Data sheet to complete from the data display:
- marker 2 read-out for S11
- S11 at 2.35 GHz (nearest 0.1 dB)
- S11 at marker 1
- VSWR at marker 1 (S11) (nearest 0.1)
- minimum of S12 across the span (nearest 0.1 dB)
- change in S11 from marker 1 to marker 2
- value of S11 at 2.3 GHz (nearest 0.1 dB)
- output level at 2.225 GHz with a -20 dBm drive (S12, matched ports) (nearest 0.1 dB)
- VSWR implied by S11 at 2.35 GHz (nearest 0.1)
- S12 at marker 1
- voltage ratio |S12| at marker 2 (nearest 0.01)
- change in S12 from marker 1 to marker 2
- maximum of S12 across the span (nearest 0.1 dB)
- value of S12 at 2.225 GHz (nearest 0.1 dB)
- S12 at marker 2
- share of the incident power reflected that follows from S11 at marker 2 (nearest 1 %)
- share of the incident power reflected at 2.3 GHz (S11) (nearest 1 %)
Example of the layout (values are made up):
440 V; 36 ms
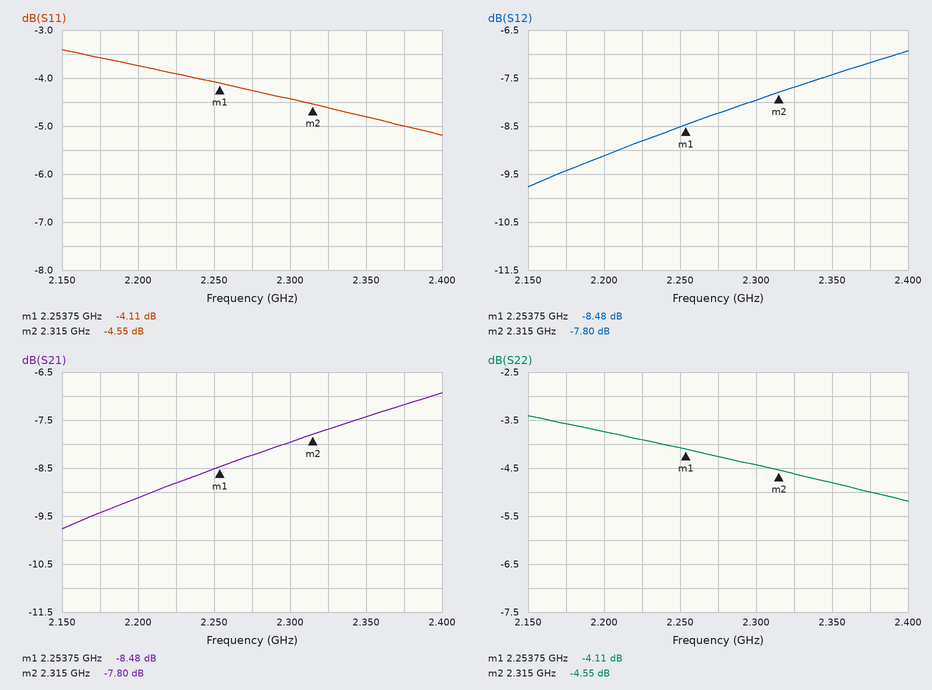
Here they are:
-4.55 dB; -4.8 dB; -4.11 dB; 4.3; -9.8 dB; -0.44 dB; -4.4 dB; -28.8 dBm; 3.7; -8.48 dB; 0.41; 0.68 dB; -6.9 dB; -8.8 dB; -7.80 dB; 35 %; 36 %
